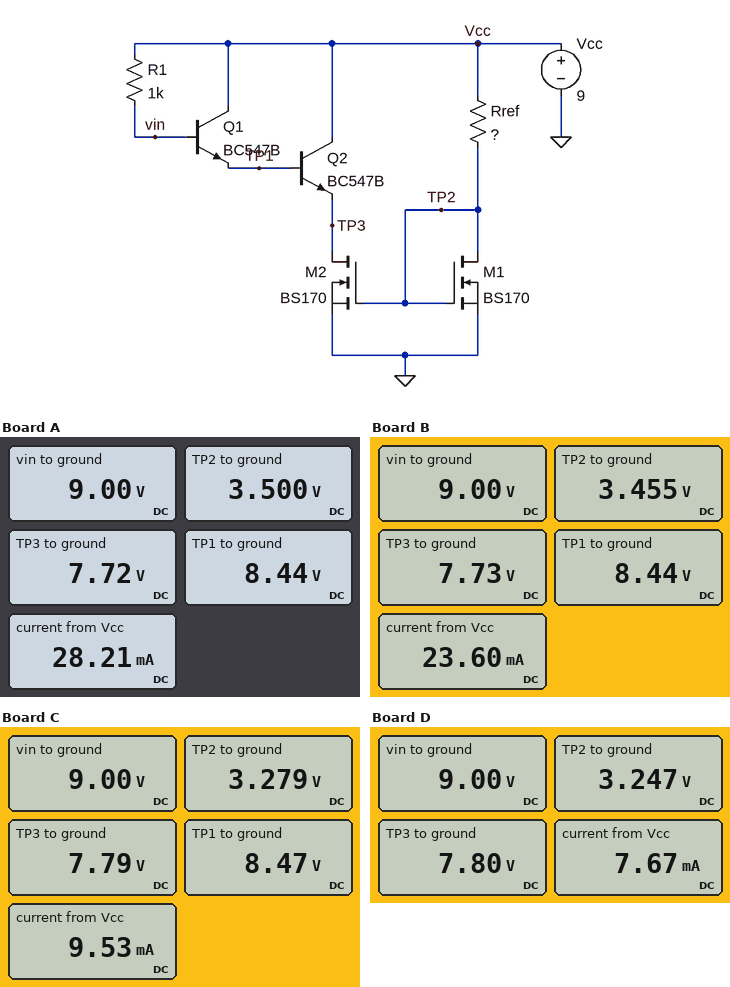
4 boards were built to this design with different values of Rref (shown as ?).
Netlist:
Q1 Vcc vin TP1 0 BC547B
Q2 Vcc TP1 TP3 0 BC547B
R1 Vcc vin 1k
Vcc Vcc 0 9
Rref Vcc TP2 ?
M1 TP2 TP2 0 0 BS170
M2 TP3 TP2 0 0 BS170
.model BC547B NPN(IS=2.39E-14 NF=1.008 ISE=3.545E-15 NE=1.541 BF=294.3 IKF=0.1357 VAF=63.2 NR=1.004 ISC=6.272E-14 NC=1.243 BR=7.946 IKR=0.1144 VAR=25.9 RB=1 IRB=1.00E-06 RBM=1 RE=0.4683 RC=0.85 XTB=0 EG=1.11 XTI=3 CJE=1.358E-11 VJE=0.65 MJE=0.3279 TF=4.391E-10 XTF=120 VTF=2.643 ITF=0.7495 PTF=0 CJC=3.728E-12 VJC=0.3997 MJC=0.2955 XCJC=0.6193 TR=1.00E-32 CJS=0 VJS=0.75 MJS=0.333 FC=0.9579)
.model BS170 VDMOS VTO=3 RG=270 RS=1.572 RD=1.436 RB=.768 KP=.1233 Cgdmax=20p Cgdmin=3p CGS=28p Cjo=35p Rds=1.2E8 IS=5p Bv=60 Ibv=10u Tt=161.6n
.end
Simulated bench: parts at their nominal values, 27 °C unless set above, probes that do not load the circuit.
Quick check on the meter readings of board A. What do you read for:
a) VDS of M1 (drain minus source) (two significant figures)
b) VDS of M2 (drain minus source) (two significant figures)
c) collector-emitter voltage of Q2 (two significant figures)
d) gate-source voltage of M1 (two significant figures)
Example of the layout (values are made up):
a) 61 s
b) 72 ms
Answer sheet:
a) 3.5 V
b) 7.7 V
c) 1.3 V
d) 3.5 V
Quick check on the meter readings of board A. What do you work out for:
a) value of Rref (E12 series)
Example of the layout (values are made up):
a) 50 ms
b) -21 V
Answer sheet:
a) 390 Ω
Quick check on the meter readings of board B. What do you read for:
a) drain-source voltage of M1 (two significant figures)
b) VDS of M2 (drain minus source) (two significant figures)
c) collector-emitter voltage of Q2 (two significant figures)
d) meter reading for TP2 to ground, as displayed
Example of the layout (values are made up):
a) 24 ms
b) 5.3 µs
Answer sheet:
a) 3.5 V
b) 7.7 V
c) 1.3 V
d) 3.455 V
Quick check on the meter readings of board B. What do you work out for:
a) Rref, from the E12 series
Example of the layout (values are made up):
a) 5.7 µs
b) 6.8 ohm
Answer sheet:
a) 470 Ω
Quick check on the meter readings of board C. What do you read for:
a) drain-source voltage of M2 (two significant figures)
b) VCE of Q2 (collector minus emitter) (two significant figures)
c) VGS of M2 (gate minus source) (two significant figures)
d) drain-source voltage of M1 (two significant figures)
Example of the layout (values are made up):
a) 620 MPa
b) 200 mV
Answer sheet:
a) 7.8 V
b) 1.2 V
c) 3.3 V
d) 3.3 V
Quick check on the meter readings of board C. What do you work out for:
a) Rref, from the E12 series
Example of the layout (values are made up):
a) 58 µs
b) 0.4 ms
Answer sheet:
a) 1.2 kΩ
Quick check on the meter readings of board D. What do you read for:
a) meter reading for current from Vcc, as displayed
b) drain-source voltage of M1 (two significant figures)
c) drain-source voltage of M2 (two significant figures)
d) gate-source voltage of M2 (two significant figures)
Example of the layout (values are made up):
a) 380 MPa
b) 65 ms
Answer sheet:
a) 7.67 mA
b) 3.2 V
c) 7.8 V
d) 3.2 V
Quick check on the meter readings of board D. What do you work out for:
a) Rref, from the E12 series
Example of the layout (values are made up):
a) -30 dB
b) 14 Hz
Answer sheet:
a) 1.5 kΩ
